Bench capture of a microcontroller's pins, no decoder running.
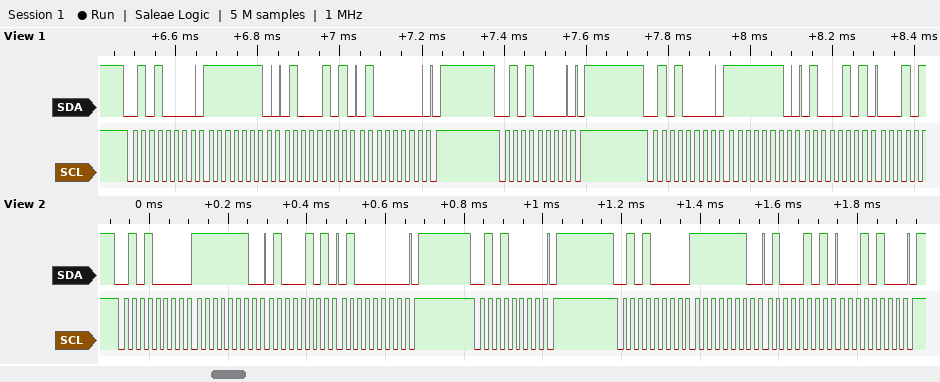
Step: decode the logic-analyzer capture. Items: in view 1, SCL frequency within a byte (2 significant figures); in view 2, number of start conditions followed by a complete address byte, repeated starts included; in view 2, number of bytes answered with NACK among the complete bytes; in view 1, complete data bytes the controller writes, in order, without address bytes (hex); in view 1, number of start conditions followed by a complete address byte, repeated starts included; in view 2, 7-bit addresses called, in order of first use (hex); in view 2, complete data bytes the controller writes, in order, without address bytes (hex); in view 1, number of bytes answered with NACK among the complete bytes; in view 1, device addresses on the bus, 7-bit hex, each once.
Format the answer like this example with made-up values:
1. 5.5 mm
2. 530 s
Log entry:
1. 50 kHz
2. 3
3. 0
4. FE 45 40 FE 45
5. 3
6. 0x28
7. FE 45 40 FE 45 14
8. 0
9. 0x28
